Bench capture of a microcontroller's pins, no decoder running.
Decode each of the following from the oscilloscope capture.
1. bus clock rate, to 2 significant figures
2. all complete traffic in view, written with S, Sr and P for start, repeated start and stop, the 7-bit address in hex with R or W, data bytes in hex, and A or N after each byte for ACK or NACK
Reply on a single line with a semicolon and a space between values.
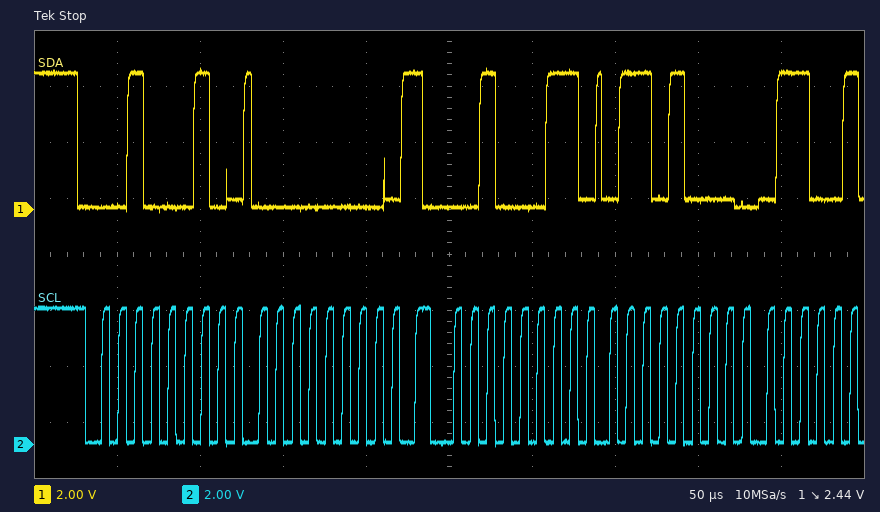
100 kHz; S 11W A 00 A Sr 11R A 68 A
